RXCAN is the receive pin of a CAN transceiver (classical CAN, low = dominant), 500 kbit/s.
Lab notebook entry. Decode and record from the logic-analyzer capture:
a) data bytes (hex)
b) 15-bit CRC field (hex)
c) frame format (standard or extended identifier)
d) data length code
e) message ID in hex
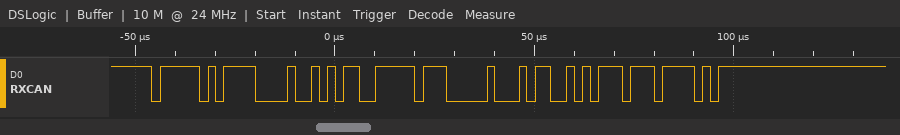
AC FF 00 B2
0x5DDE
standard
4
0x7EF
